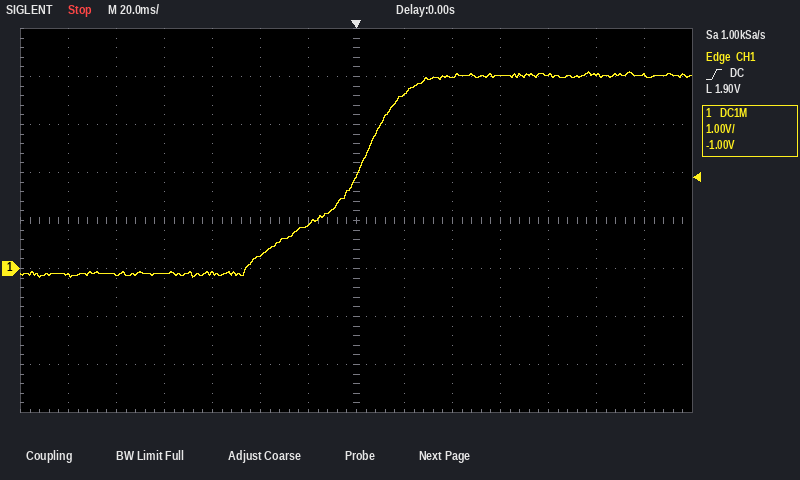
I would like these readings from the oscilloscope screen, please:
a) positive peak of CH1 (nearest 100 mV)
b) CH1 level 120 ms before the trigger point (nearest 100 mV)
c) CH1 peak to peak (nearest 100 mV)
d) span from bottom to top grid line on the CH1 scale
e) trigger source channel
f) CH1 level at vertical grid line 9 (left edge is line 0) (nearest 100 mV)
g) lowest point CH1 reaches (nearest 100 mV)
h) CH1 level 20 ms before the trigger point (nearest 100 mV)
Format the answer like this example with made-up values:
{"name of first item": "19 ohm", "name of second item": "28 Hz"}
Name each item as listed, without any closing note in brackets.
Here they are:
{"positive peak of CH1": "4.1 V", "CH1 level 120 ms before the trigger point": "-100 mV", "CH1 peak to peak": "4.3 V", "span from bottom to top grid line on the CH1 scale": "8 V", "trigger source channel": "CH1", "CH1 level at vertical grid line 9 (left edge is line 0)": "4.0 V", "lowest point CH1 reaches": "-200 mV", "CH1 level 20 ms before the trigger point": "900 mV"}
